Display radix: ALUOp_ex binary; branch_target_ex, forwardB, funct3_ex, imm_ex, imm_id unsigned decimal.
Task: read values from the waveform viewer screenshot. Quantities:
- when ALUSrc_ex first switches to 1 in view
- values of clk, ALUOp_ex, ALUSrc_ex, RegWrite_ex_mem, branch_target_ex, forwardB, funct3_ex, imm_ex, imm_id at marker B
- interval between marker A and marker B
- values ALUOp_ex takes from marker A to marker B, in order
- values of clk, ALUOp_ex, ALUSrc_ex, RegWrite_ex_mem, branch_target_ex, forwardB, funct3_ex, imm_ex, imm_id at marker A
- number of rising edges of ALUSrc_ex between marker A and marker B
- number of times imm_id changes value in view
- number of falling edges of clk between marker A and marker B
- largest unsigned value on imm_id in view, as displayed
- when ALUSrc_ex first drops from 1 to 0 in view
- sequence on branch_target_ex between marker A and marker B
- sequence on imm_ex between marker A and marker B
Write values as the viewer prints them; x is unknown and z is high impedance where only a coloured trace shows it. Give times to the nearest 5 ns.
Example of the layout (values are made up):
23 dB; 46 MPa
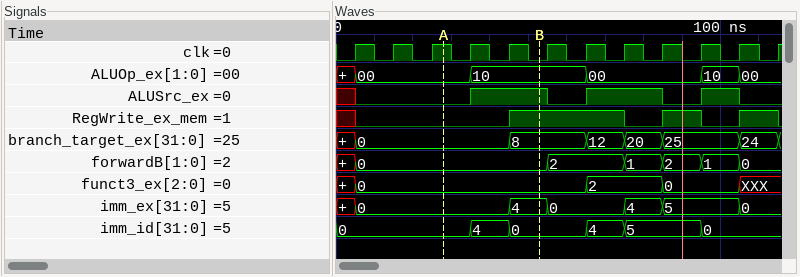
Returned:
35 ns; clk=0, ALUOp_ex=10, ALUSrc_ex=1, RegWrite_ex_mem=1, branch_target_ex=8, forwardB=0, funct3_ex=0, imm_ex=4, imm_id=0; 25 ns; 00, 10; clk=1, ALUOp_ex=00, ALUSrc_ex=0, RegWrite_ex_mem=0, branch_target_ex=0, forwardB=0, funct3_ex=0, imm_ex=0, imm_id=0; 1; 5; 3; 5; 55 ns; 0, 8; 0, 4
